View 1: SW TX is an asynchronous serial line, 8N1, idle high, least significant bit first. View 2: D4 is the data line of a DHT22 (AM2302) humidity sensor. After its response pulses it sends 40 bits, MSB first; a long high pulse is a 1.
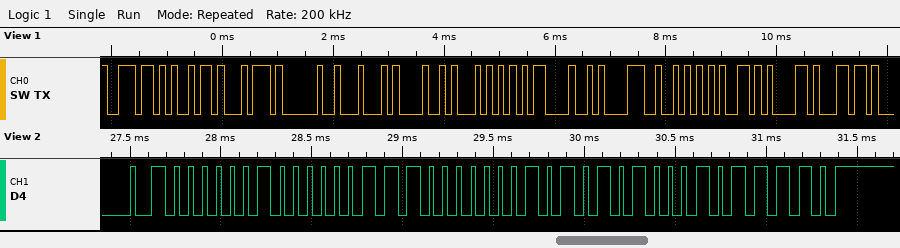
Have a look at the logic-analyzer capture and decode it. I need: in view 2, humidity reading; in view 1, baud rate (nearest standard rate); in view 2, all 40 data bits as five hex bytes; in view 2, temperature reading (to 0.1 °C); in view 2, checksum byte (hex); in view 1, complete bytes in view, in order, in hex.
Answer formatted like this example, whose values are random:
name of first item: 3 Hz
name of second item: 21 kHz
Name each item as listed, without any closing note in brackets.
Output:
in view 2, humidity reading: 51.9 %
in view 1, baud rate: 9600 baud
in view 2, all 40 data bits as five hex bytes: 02 07 01 54 5E
in view 2, temperature reading: 34.0 °C
in view 2, checksum byte: 0x5E
in view 1, complete bytes in view, in order, in hex: 6E 69 74 20 44 48 54 0D 0A 52 65 61 6C
